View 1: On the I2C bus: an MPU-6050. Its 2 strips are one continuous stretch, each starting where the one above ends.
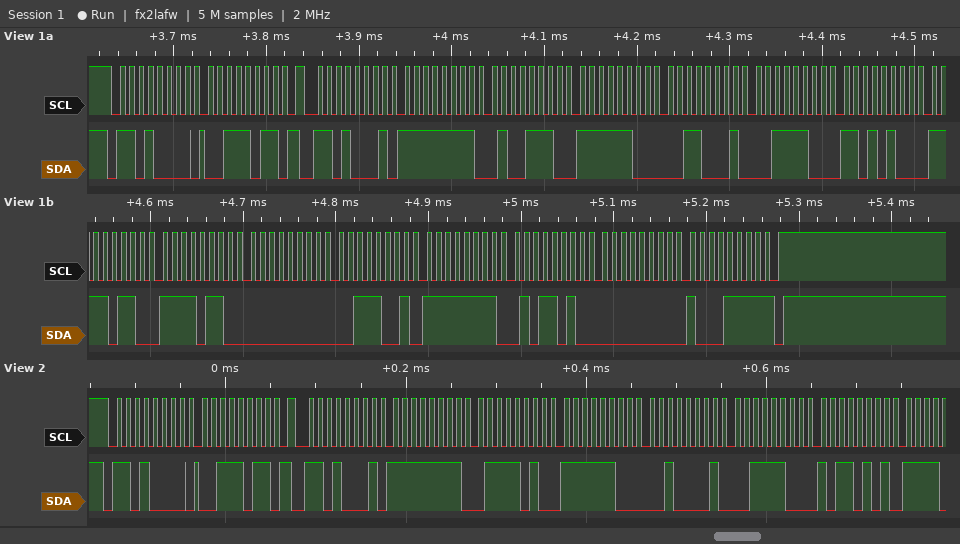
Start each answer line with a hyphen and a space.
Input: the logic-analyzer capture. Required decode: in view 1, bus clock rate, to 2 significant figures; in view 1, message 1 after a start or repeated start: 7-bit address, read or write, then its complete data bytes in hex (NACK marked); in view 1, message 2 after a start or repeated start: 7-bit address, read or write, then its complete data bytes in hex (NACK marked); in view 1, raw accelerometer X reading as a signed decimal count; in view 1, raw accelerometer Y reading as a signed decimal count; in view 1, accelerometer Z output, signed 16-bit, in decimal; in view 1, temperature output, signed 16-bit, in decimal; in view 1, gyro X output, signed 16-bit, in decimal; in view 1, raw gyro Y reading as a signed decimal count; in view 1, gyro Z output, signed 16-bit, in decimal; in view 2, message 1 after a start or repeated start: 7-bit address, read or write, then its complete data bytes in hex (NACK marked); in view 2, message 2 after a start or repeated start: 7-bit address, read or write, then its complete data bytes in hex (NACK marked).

- 100 kHz
- 0x68 write: 3B
- 0x68 read: FF 4E FC 31 3C D4 F6 F6 00 39 FF 5A 00 8F NACK
- -178
- -975
- 15572
- -2314
- 57
- -166
- 143
- 0x68 write: 3B
- 0x68 read: FF 7A FC 21 3C B5
